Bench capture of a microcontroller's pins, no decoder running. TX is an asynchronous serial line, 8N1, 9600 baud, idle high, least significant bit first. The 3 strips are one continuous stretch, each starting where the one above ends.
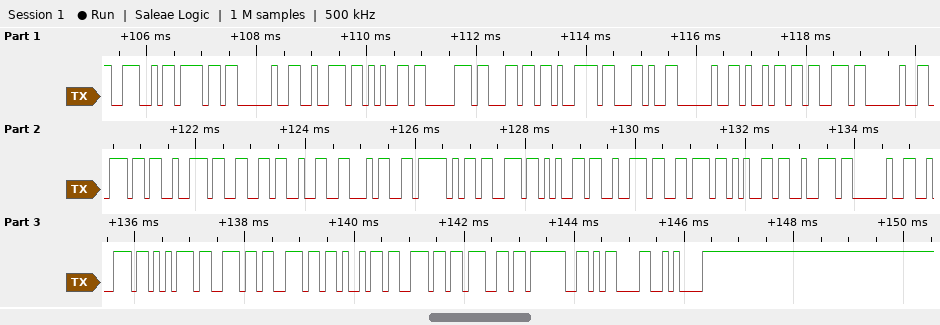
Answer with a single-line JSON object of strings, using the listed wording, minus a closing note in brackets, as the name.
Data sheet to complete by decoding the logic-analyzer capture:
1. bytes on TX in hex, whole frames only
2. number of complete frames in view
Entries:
{"bytes on TX in hex, whole frames only": "4E 6F 20 72 65 70 6C 79 2C 20 69 73 20 6E 72 66 32 34 5F 73 65 72 76 65 72 20 72 75 6E 6E 69 6E 67 3F 0D 0A", "number of complete frames in view": "36"}
